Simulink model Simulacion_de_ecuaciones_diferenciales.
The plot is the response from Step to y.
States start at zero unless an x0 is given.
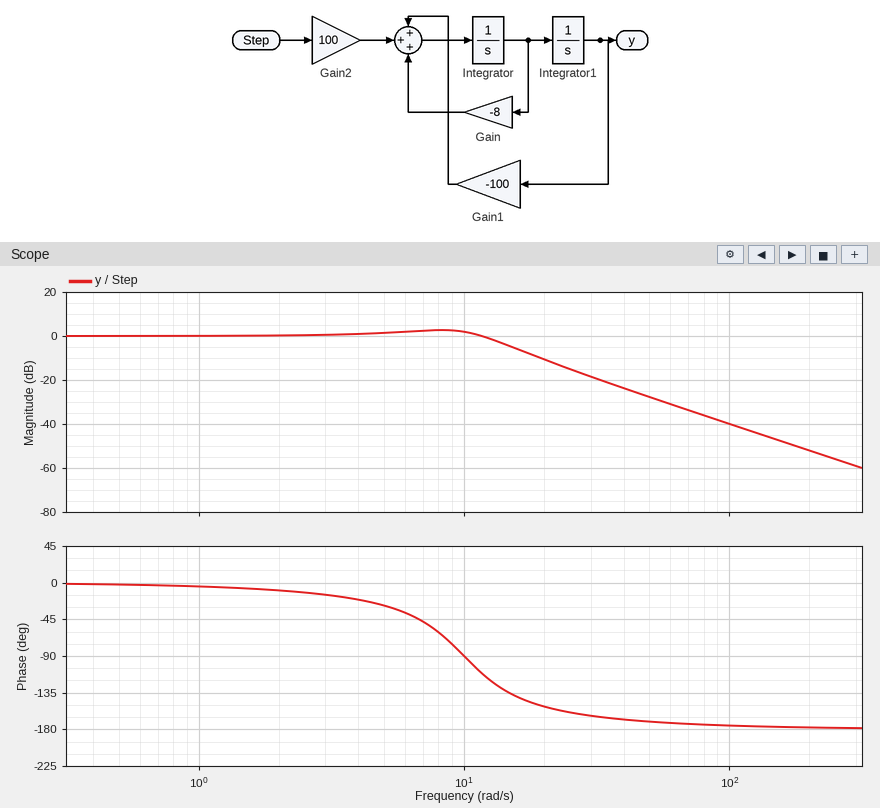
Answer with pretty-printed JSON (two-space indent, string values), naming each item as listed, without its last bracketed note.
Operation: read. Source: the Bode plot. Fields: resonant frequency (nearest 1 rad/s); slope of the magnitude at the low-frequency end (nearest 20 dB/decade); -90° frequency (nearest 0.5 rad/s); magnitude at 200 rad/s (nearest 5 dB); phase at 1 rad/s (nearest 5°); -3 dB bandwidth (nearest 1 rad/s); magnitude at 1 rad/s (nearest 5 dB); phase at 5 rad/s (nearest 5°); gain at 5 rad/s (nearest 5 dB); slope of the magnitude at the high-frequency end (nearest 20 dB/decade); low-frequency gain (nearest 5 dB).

{
  "resonant frequency": "8 rad/s",
  "slope of the magnitude at the low-frequency end": "0 dB/decade",
  "-90° frequency": "10.0 rad/s",
  "magnitude at 200 rad/s": "-50 dB",
  "phase at 1 rad/s": "-5°",
  "-3 dB bandwidth": "14 rad/s",
  "magnitude at 1 rad/s": "0 dB",
  "phase at 5 rad/s": "-30°",
  "gain at 5 rad/s": "0 dB",
  "slope of the magnitude at the high-frequency end": "-40 dB/decade",
  "low-frequency gain": "0 dB"
}
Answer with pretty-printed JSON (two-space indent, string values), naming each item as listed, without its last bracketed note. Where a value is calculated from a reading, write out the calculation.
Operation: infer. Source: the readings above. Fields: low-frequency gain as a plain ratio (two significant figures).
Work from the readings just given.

{
  "low-frequency gain as a plain ratio": "10^(0 / 20) = 1.0"
}
